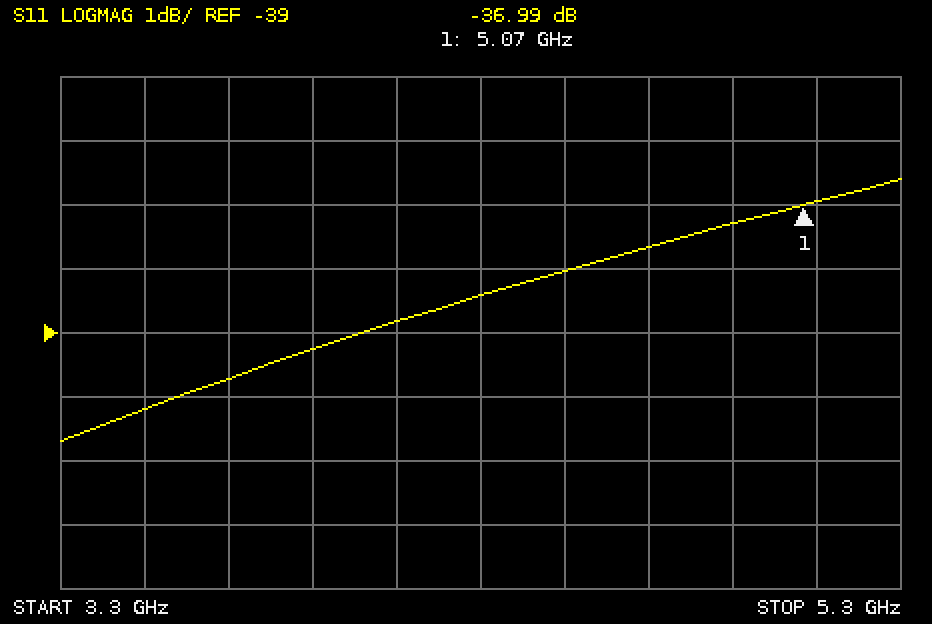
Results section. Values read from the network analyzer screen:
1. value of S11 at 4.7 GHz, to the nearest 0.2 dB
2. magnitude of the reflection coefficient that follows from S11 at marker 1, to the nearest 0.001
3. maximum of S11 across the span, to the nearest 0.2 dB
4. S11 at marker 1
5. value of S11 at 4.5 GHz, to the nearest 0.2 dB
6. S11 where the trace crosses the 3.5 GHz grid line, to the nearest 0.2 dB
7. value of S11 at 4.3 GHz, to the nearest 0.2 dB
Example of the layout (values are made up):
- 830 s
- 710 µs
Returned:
- -37.6 dB
- 0.014
- -36.6 dB
- -36.99 dB
- -38.0 dB
- -40.2 dB
- -38.4 dB
